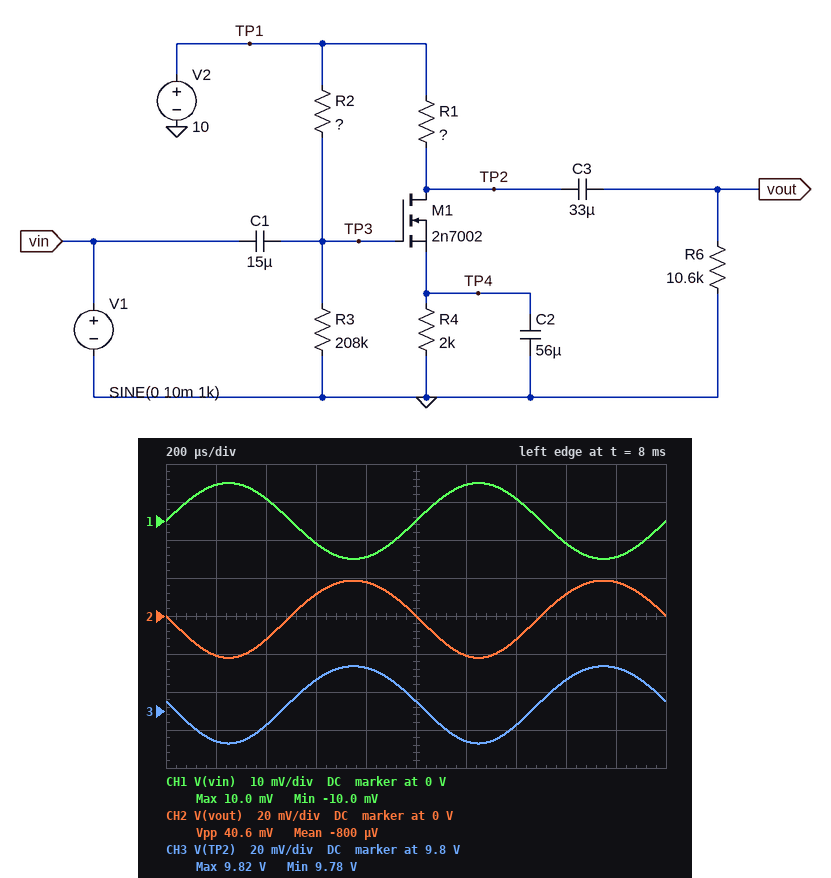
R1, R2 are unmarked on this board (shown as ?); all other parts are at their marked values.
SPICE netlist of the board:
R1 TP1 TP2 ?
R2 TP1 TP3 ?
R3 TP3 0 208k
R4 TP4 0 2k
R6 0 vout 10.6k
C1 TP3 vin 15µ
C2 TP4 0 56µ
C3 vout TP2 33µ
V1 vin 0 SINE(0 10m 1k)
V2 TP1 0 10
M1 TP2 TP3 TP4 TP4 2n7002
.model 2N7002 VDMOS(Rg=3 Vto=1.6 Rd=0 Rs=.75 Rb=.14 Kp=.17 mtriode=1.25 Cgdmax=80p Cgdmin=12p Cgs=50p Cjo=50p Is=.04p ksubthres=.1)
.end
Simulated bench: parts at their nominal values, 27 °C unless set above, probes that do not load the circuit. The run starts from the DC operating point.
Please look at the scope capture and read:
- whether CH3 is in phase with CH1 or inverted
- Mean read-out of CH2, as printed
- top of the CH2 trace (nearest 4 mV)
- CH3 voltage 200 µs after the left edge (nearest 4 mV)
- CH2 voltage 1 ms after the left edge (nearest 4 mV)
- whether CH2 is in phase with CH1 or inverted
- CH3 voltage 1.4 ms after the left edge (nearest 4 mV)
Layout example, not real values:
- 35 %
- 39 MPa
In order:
- inverted
- -800 µV
- 20 mV
- 9.784 V
- 0 V
- inverted
- 9.792 V
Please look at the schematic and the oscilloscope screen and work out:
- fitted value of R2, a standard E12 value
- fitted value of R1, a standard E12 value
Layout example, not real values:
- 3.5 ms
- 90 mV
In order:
- 1.2 MΩ
- 8.2 kΩ
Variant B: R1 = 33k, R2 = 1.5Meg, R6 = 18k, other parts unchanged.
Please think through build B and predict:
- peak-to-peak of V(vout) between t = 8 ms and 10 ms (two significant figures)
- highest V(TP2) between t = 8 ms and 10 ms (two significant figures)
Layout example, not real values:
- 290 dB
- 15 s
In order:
- 1.8 mV
- 10 V
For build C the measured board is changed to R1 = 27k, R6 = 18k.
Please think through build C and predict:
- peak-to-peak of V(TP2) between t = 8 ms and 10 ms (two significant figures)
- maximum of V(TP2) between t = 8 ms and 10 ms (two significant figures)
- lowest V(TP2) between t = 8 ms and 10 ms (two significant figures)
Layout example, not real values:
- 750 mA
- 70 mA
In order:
- 95 mV
- 9.4 V
- 9.3 V
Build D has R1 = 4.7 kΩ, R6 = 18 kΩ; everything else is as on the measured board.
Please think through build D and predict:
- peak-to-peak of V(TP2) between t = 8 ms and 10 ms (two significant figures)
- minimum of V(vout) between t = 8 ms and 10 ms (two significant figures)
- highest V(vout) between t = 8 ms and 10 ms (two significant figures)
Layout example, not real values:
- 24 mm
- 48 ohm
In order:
- 33 mV
- -18 mV
- 15 mV
